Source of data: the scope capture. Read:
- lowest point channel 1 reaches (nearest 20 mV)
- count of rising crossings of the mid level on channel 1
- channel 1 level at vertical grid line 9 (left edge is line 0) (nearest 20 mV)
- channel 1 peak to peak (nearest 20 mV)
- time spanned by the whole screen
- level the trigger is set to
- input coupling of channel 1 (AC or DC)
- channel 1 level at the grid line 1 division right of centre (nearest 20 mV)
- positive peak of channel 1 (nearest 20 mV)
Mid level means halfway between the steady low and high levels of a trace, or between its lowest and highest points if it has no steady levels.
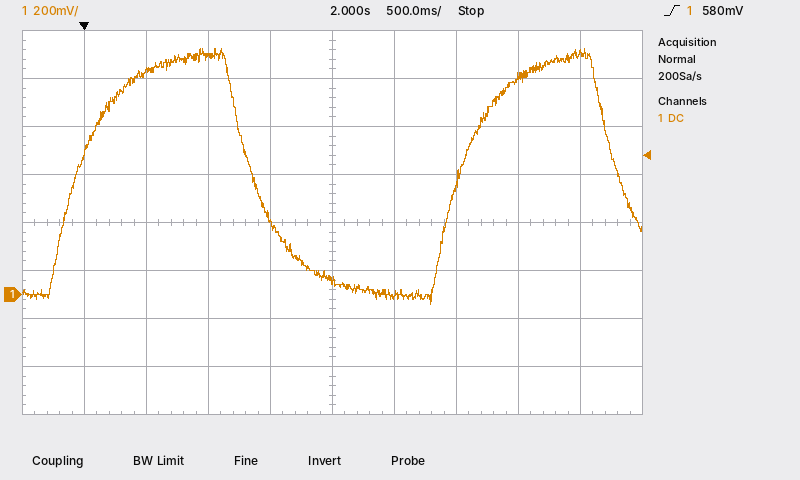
-40 mV
2
1.00 V
1.06 V
5 s
580 mV
DC
0 mV
1.02 V
